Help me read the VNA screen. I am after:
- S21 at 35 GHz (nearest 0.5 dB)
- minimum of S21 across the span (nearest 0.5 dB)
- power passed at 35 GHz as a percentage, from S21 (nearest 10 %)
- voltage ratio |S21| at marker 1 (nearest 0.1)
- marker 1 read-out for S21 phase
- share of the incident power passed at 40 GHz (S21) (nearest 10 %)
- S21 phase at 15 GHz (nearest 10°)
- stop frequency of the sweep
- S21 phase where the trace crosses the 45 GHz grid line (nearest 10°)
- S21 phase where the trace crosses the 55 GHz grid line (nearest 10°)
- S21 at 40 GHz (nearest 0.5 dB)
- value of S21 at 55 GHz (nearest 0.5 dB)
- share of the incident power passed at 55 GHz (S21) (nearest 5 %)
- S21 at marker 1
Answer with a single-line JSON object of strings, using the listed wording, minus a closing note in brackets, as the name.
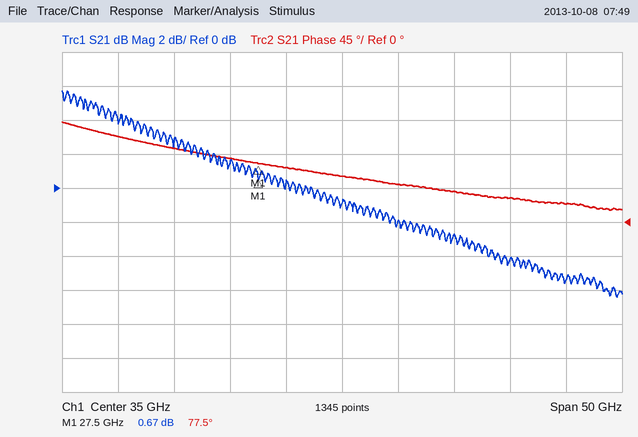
{"S21 at 35 GHz": "-1.0 dB", "minimum of S21 across the span": "-6.5 dB", "power passed at 35 GHz as a percentage, from S21": "80 %", "voltage ratio |S21| at marker 1": "1.1", "marker 1 read-out for S21 phase": "77.5°", "share of the incident power passed at 40 GHz (S21)": "60 %", "S21 phase at 15 GHz": "110°", "stop frequency of the sweep": "60 GHz", "S21 phase where the trace crosses the 45 GHz grid line": "40°", "S21 phase where the trace crosses the 55 GHz grid line": "20°", "S21 at 40 GHz": "-2.0 dB", "value of S21 at 55 GHz": "-5.5 dB", "share of the incident power passed at 55 GHz (S21)": "30 %", "S21 at marker 1": "0.67 dB"}
